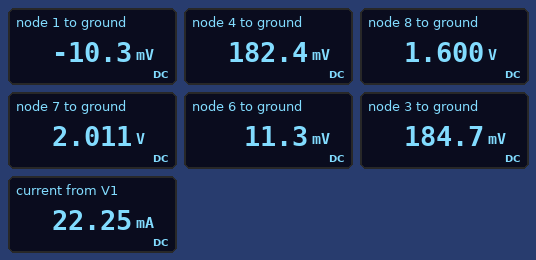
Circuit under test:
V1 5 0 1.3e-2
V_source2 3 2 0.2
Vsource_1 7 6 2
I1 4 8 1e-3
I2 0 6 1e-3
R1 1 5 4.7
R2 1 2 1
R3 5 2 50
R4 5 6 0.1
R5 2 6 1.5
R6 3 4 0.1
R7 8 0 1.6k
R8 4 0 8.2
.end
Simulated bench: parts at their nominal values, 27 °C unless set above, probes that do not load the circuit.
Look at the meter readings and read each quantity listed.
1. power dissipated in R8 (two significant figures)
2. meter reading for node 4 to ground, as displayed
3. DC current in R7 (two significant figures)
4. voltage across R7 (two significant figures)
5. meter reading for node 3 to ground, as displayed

4.1 mW
182.4 mV
1.0 mA
1.6 V
184.7 mV
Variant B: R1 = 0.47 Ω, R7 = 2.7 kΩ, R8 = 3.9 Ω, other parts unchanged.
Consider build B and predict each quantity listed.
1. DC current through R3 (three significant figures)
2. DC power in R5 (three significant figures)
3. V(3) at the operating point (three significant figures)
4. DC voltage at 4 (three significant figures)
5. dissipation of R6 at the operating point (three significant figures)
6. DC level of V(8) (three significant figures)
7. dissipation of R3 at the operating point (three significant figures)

688 µA
697 µW
179 mV
174 mV
208 µW
2.70 V
23.6 µW
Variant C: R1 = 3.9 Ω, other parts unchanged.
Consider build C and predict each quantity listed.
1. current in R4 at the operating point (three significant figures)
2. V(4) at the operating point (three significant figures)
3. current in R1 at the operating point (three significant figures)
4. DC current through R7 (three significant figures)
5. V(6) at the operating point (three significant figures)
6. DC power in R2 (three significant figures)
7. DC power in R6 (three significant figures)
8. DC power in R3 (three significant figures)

16.2 mA
183 mV
5.60 mA
1.00 mA
11.4 mV
31.3 µW
54.5 µW
15.0 µW
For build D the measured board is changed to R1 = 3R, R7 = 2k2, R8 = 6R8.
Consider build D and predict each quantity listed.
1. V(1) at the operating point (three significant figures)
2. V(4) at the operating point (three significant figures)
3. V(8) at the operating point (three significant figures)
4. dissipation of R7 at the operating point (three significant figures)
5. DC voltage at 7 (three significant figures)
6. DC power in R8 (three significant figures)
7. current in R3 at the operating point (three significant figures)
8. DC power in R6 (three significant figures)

-9.93 mV
180 mV
2.20 V
2.20 mW
2.01 V
4.75 mW
611 µA
75.2 µW
